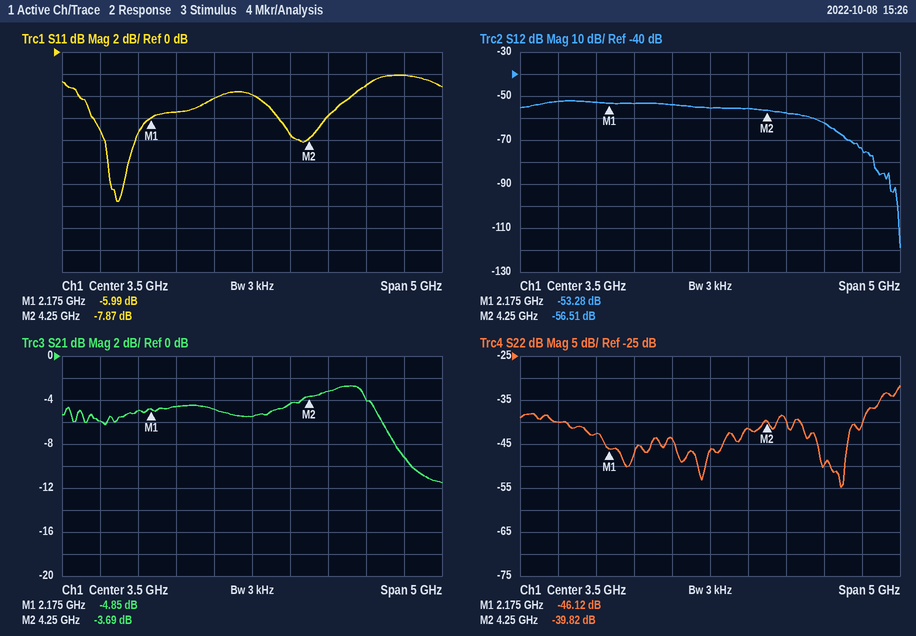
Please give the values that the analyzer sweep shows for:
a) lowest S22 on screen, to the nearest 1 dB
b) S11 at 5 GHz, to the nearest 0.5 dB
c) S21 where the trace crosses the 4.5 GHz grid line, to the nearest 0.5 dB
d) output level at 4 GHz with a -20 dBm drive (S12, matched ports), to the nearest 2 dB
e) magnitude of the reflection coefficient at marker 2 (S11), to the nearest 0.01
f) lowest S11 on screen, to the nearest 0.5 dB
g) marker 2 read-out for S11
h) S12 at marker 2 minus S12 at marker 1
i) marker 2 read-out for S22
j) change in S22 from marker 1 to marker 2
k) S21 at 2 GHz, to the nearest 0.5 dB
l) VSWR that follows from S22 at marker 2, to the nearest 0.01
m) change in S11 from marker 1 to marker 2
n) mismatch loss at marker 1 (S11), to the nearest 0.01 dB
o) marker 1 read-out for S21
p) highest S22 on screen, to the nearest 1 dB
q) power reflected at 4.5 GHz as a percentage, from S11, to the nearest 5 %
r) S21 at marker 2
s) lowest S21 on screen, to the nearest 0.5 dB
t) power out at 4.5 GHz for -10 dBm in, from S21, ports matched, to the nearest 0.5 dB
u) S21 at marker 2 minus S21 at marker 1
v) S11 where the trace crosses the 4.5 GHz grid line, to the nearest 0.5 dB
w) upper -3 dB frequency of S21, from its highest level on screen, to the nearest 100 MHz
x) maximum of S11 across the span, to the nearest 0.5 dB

-55 dB
-3.0 dB
-3.0 dB
-76 dBm
0.40
-13.5 dB
-7.87 dB
-3.23 dB
-39.82 dB
6.30 dB
-5.0 dB
1.02
-1.88 dB
1.26 dB
-4.85 dB
-32 dB
25 %
-3.69 dB
-11.5 dB
-13.0 dBm
1.16 dB
-6.0 dB
5.2 GHz
-2.0 dB
